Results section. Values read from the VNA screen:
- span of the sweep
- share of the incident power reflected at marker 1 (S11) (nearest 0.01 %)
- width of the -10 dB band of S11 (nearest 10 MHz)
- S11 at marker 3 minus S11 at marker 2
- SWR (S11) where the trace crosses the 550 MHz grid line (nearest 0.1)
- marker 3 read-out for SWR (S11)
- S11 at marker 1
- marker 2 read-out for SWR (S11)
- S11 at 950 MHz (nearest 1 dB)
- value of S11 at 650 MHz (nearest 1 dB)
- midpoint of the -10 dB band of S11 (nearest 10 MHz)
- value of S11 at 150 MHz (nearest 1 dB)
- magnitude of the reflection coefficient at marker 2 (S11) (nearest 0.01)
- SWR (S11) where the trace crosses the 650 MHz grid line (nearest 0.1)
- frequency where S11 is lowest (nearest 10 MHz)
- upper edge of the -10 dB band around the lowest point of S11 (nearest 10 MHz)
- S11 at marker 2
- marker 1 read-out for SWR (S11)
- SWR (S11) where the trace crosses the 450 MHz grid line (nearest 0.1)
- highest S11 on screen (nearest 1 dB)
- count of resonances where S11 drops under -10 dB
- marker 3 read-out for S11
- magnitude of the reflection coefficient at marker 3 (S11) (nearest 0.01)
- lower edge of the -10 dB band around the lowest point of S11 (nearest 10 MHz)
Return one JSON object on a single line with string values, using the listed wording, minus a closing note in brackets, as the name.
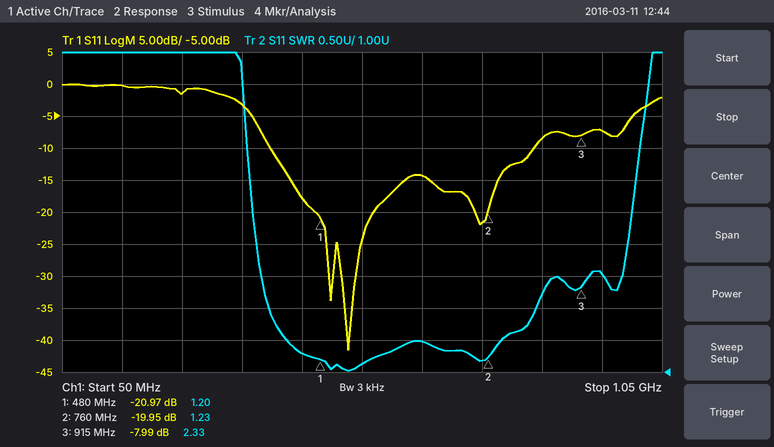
{"span of the sweep": "1 GHz", "share of the incident power reflected at marker 1 (S11)": "0.80 %", "width of the -10 dB band of S11": "440 MHz", "S11 at marker 3 minus S11 at marker 2": "11.96 dB", "SWR (S11) where the trace crosses the 550 MHz grid line": "1.1", "marker 3 read-out for SWR": "2.33", "S11 at marker 1": "-20.97 dB", "marker 2 read-out for SWR": "1.23", "S11 at 950 MHz": "-7 dB", "value of S11 at 650 MHz": "-14 dB", "midpoint of the -10 dB band of S11": "620 MHz", "value of S11 at 150 MHz": "0 dB", "magnitude of the reflection coefficient at marker 2 (S11)": "0.10", "SWR (S11) where the trace crosses the 650 MHz grid line": "1.5", "frequency where S11 is lowest": "530 MHz", "upper edge of the -10 dB band around the lowest point of S11": "840 MHz", "S11 at marker 2": "-19.95 dB", "marker 1 read-out for SWR": "1.20", "SWR (S11) where the trace crosses the 450 MHz grid line": "1.3", "highest S11 on screen": "0 dB", "count of resonances where S11 drops under -10 dB": "3", "marker 3 read-out for S11": "-7.99 dB", "magnitude of the reflection coefficient at marker 3 (S11)": "0.40", "lower edge of the -10 dB band around the lowest point of S11": "400 MHz"}
